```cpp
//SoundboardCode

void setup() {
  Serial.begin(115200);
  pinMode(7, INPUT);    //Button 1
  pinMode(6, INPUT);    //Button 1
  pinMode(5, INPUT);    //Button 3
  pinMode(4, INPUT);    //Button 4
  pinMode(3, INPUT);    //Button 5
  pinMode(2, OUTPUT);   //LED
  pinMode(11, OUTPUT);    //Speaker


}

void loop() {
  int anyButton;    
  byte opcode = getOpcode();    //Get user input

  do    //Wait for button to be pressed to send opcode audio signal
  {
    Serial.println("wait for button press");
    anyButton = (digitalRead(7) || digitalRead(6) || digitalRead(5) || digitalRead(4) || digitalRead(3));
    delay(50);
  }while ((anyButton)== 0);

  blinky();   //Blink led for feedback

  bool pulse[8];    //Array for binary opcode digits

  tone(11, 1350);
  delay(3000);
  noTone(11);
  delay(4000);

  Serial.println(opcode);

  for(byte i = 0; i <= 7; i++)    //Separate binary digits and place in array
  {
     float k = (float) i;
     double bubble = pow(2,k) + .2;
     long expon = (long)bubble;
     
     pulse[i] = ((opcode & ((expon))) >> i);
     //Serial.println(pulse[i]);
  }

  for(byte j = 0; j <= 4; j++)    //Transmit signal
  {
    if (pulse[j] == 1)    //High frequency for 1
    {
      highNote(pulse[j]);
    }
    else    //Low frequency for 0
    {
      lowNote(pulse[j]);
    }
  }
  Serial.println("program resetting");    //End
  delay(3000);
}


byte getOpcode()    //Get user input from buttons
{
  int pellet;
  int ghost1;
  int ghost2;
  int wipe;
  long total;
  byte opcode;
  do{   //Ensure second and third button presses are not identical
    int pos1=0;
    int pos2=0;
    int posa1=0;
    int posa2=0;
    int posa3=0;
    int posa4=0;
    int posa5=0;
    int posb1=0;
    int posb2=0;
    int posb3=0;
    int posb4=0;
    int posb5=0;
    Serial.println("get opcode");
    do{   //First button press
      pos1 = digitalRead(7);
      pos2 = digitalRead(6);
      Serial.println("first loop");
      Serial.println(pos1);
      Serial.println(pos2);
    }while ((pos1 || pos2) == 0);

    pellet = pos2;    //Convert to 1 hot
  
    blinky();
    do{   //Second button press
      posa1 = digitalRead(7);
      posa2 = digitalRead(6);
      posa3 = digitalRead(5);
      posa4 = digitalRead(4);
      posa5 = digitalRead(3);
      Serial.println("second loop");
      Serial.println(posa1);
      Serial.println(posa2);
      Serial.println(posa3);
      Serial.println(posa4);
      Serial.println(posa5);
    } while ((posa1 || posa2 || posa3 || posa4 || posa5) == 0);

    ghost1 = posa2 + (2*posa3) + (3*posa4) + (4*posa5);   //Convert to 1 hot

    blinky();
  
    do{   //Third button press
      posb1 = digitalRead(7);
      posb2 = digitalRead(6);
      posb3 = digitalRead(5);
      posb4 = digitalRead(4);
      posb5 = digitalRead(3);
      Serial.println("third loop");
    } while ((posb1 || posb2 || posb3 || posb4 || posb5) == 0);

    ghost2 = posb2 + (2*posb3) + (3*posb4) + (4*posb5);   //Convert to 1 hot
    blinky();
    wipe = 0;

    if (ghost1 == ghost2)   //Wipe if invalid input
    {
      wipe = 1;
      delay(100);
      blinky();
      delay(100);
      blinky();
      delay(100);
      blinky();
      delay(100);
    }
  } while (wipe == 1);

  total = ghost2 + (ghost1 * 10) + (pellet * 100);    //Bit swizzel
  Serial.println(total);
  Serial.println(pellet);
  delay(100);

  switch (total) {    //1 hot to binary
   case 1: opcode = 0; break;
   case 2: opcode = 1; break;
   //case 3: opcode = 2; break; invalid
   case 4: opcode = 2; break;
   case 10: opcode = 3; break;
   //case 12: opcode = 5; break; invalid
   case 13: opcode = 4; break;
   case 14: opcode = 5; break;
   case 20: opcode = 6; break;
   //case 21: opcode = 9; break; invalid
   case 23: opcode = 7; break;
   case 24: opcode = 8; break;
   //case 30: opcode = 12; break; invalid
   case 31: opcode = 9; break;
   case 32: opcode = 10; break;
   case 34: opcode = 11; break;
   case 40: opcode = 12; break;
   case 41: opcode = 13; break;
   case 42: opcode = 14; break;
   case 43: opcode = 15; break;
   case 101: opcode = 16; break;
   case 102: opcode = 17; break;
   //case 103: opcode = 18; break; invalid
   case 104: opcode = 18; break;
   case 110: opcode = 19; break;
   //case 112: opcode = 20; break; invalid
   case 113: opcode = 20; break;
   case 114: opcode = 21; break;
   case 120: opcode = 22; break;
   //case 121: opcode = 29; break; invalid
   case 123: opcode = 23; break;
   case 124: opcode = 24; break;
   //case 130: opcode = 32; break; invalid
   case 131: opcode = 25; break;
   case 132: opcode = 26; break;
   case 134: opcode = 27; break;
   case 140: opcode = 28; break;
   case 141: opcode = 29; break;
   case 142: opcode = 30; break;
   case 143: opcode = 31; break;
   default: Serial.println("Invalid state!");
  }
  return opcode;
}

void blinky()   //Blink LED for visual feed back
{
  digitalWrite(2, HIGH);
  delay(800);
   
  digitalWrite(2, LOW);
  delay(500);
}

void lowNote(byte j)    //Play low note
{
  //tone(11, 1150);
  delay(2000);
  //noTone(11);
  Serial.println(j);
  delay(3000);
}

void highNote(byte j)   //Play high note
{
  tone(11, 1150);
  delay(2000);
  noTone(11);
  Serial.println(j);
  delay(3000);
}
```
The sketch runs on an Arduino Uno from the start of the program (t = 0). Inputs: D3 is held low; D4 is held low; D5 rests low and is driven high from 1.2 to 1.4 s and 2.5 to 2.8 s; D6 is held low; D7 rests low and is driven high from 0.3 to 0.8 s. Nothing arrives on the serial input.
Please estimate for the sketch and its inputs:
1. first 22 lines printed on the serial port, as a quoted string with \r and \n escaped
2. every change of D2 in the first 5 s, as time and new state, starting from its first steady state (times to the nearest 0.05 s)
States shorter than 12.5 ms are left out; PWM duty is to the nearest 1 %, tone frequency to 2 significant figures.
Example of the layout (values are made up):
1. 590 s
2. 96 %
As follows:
1. "get opcode\r\nfirst loop\r\n0\r\n0\r\nfirst loop\r\n0\r\n0\r\nfirst loop\r\n0\r\n0\r\nfirst loop\r\n0\r\n0\r\nfirst loop\r\n0\r\n0\r\nfirst loop\r\n0\r\n0\r\nfirst loop\r\n0\r\n0\r\n"
2. 0 s low; 0.3 s high; 1.1 s low; 2.5 s high; 3.3 s low
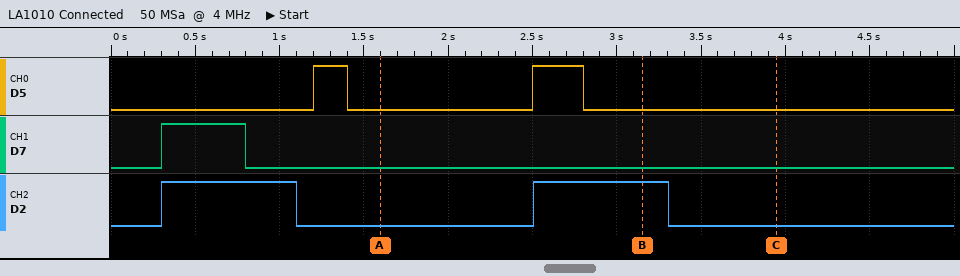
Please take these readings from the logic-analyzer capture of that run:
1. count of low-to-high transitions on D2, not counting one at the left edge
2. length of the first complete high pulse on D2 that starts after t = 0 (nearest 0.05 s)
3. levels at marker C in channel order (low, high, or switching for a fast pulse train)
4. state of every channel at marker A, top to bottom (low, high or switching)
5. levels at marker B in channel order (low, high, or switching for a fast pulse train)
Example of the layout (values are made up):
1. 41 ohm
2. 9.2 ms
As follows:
1. 2
2. 0.80 s
3. D5 low, D7 low, D2 low
4. D5 low, D7 low, D2 low
5. D5 low, D7 low, D2 high
